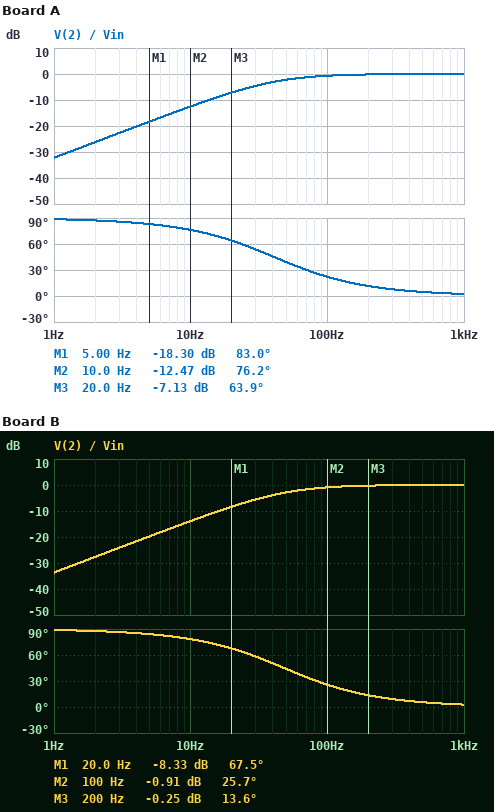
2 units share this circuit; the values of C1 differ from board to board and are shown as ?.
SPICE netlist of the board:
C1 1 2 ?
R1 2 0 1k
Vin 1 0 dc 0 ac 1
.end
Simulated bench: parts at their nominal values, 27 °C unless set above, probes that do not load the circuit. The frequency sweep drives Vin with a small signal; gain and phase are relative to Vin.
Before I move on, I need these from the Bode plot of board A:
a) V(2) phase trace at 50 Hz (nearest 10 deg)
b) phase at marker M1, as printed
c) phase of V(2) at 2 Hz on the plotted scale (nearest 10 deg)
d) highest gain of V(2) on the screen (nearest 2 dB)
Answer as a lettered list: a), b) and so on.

a) 40 deg
b) 83.0 deg
c) 90 deg
d) 0 dB
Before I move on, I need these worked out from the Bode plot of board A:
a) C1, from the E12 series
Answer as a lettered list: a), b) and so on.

a) 3.9 µF
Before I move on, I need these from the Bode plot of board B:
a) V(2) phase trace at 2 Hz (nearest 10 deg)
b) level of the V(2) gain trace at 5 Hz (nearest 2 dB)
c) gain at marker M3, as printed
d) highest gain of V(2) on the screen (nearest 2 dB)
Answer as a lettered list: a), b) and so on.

a) 90 deg
b) -20 dB
c) -0.25 dB
d) 0 dB
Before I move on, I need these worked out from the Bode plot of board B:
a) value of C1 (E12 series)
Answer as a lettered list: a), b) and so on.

a) 3.3 µF
